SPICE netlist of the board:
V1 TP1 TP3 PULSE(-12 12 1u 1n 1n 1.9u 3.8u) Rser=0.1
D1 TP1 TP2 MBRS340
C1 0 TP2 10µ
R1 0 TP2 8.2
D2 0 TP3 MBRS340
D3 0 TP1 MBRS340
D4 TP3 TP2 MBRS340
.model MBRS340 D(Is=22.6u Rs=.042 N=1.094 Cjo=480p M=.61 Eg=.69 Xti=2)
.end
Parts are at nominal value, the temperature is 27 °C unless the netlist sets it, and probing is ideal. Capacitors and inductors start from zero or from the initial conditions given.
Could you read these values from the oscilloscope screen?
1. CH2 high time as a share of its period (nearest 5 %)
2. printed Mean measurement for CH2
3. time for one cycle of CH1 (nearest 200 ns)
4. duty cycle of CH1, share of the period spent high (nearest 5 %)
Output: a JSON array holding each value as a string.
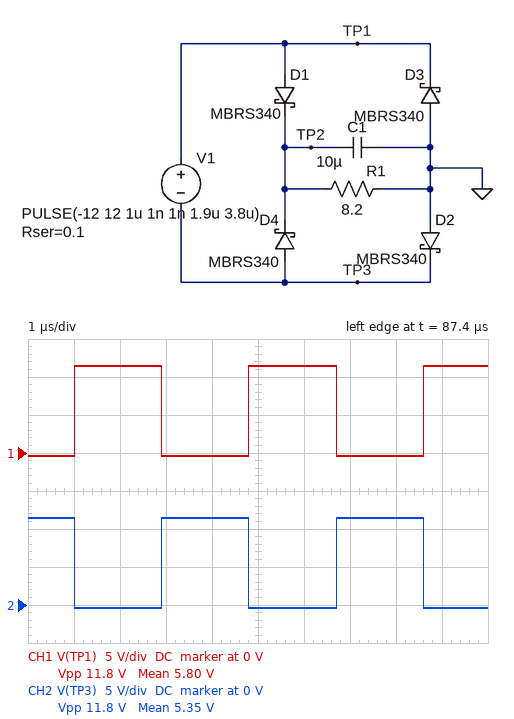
["50 %", "5.35 V", "3.8 µs", "50 %"]
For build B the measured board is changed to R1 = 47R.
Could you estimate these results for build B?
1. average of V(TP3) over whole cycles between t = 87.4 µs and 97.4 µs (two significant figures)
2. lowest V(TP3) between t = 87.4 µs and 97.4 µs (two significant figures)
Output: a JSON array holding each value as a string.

["5.7 V", "-270 mV"]
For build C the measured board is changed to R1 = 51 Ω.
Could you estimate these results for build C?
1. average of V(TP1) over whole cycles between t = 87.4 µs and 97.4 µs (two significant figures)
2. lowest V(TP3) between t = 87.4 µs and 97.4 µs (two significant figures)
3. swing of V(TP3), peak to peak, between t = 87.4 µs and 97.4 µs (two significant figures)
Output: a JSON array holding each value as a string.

["5.7 V", "-270 mV", "12 V"]
